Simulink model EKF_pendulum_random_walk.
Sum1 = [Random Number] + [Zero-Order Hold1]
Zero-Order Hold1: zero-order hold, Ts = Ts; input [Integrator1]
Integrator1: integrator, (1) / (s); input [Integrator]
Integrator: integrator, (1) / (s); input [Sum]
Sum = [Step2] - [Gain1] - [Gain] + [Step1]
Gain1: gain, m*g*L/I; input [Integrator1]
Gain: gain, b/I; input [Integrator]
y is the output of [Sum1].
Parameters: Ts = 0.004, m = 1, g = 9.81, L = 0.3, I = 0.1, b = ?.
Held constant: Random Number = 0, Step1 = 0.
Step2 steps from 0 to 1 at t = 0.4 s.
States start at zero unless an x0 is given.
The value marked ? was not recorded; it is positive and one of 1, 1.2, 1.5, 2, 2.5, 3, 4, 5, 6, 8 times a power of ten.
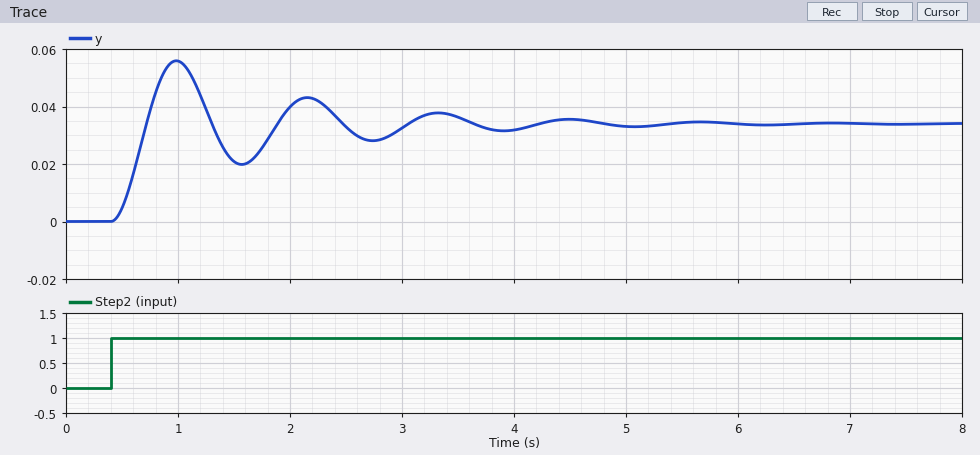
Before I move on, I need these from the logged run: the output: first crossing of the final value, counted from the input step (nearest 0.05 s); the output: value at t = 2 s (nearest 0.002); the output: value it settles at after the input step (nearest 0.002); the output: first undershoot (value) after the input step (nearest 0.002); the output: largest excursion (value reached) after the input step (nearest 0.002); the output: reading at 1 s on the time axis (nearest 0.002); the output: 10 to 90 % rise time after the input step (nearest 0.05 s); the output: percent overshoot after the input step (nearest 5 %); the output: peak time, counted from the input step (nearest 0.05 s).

0.30 s
0.040
0.034
0.020
0.056
0.056
0.20 s
65 %
0.60 s
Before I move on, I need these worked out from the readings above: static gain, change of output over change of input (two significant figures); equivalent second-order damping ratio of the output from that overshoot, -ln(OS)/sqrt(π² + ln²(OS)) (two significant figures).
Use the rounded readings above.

0.034
0.14
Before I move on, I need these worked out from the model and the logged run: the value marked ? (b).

0.15
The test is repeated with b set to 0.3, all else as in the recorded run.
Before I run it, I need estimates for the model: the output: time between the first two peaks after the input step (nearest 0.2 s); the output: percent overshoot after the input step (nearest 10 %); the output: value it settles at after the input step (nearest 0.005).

1.2 s
40 %
0.035
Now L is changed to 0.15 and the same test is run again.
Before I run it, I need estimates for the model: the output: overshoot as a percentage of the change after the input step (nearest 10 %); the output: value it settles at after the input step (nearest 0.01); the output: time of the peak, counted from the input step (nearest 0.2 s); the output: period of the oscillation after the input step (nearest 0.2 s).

50 %
0.07
0.8 s
1.6 s
